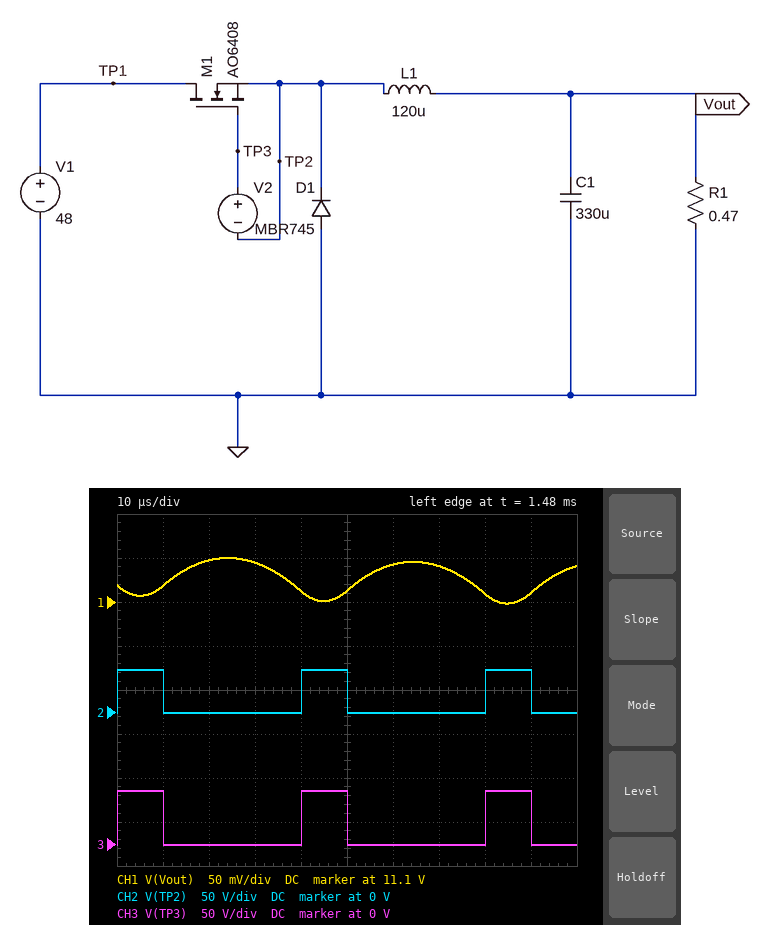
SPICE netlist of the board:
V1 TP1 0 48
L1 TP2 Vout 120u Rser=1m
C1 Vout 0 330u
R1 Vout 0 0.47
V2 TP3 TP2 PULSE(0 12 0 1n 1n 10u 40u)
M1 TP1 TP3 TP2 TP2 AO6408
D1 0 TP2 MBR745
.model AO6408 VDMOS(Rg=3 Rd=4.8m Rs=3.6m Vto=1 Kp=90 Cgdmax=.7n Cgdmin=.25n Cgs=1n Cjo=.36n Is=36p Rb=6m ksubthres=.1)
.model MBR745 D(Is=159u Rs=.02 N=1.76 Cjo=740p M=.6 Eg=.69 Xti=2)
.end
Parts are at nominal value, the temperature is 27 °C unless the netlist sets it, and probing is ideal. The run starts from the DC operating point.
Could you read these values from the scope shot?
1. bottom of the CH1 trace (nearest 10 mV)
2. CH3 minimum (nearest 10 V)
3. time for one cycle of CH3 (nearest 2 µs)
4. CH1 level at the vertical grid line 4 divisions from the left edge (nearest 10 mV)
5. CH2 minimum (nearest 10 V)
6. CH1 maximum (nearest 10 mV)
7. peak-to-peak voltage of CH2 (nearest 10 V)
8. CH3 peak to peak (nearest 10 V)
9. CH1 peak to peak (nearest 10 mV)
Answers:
11.10 V
0 V
40 µs
11.11 V
0 V
11.15 V
50 V
60 V
50 mV
